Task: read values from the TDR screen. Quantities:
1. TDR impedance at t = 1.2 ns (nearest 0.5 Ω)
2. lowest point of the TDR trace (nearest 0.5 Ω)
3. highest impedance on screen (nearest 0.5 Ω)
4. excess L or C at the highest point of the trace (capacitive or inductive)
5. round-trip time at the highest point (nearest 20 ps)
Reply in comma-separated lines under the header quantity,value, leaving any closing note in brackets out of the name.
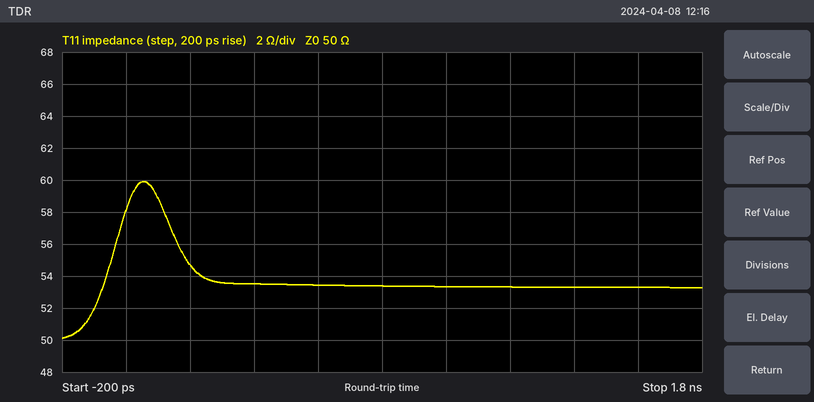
quantity,value
TDR impedance at t = 1.2 ns,53.5 Ω
lowest point of the TDR trace,50.0 Ω
highest impedance on screen,60.0 Ω
excess L or C at the highest point of the trace,inductive
round-trip time at the highest point,60 ps
